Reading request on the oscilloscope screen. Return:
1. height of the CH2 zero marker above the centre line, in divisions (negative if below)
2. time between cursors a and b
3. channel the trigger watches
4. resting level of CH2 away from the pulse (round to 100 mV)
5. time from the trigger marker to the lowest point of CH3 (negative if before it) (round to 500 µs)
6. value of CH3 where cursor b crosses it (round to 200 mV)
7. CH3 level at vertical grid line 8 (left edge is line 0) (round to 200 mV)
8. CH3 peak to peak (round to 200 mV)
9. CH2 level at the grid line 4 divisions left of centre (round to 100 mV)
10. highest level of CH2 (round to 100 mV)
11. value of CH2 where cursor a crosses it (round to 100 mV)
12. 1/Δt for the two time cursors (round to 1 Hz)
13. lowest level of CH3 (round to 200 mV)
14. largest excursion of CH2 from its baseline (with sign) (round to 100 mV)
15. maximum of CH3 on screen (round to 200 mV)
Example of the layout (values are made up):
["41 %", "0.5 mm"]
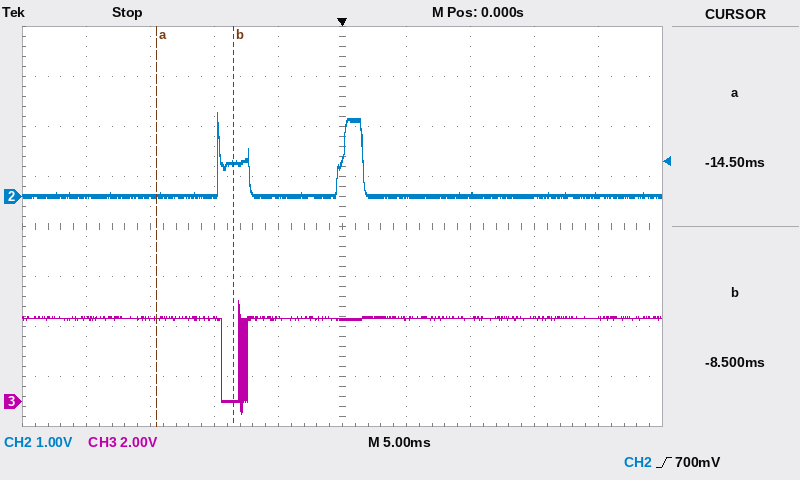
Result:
["+0.6 div", "6.0 ms", "CH2", "0.0 V", "-8.0 ms", "0.0 V", "3.4 V", "4.6 V", "0.0 V", "1.7 V", "0.0 V", "167 Hz", "-600 mV", "+1.7 V", "4.0 V"]
